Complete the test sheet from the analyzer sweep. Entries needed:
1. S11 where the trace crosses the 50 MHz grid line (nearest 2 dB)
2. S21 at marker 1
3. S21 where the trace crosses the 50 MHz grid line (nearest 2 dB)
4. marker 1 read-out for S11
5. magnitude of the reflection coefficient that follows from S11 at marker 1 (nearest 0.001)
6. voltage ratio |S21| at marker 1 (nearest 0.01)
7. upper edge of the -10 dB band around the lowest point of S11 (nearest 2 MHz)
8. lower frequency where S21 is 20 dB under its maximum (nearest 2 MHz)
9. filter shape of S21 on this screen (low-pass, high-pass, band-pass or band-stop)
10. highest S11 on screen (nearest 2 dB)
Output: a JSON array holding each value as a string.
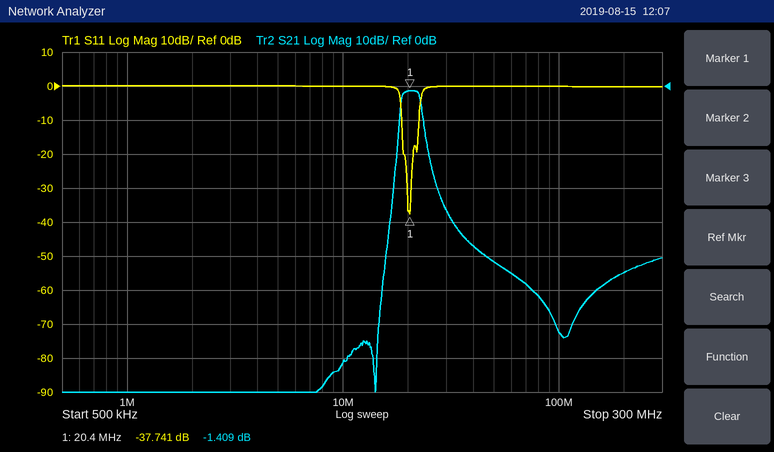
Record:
["0 dB", "-1.409 dB", "-52 dB", "-37.741 dB", "0.013", "0.85", "22 MHz", "18 MHz", "band-pass", "0 dB"]
